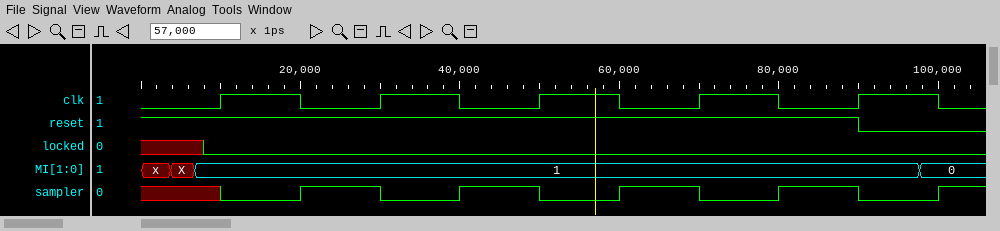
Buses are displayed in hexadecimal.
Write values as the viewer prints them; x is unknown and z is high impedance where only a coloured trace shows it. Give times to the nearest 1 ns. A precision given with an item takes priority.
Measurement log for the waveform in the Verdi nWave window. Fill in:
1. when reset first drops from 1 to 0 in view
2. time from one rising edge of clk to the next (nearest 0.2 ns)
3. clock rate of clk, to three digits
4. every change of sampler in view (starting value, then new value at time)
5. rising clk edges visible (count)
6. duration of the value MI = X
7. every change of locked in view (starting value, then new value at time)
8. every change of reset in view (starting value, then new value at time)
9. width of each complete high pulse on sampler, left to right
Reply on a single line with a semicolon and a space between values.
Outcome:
90 ns; 20 ns; 50.0 MHz; x, 0 at 10 ns, 1 at 20 ns, 0 at 30 ns, 1 at 40 ns, 0 at 50 ns, 1 at 60 ns, 0 at 70 ns, 1 at 80 ns, 0 at 90 ns, 1 at 100 ns; 5; 3 ns; x, 0 at 8 ns; 1, 0 at 90 ns; 10 ns, 10 ns, 10 ns, 10 ns
